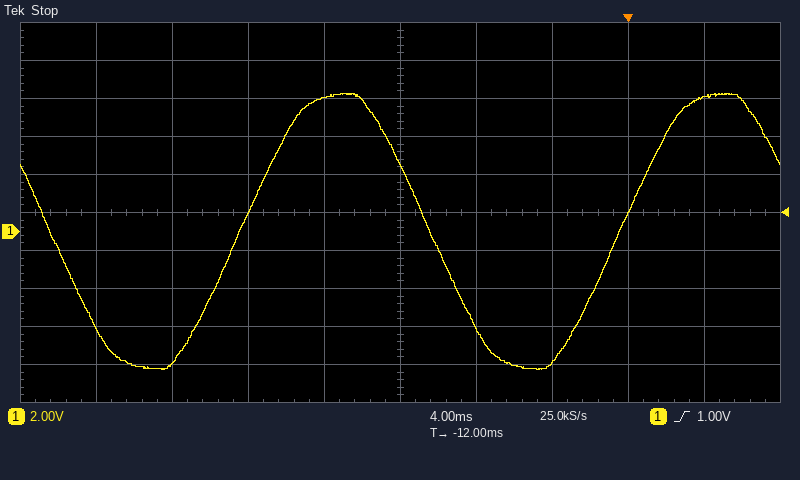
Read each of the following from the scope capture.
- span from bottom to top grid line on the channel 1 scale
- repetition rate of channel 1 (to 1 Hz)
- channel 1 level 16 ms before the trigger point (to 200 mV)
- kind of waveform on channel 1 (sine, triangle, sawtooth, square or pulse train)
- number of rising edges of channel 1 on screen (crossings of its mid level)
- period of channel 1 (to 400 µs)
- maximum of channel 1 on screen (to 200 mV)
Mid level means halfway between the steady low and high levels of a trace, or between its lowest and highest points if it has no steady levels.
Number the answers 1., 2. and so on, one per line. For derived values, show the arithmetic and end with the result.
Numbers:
1. 20 V
2. 1 / 20.0 ms ≈ 50 Hz
3. 7.0 V
4. sine
5. 2
6. 20.0 ms
7. 7.2 V
